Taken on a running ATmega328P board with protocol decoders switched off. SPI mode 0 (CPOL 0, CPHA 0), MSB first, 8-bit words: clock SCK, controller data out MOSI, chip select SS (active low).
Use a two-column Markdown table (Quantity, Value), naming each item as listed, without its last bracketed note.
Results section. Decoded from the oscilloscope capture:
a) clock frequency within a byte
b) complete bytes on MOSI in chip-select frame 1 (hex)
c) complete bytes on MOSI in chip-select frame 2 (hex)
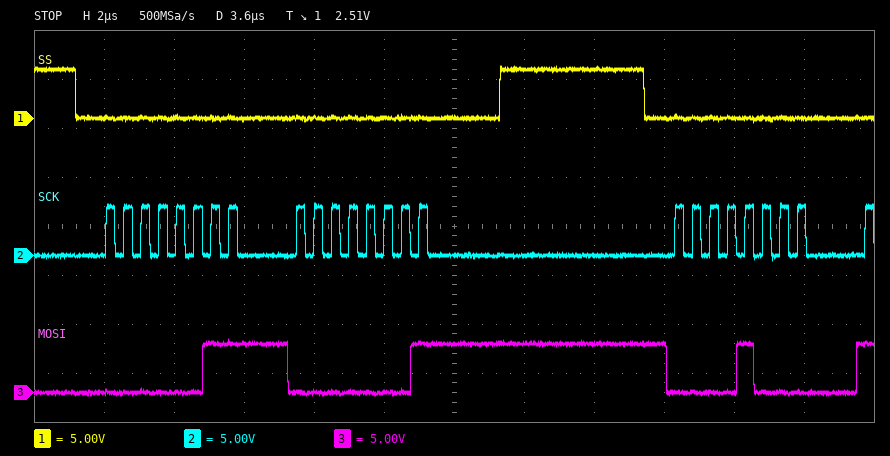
| Quantity | Value |
|---|---|
| clock frequency within a byte | 2 MHz |
| complete bytes on MOSI in chip-select frame 1 | 03 01 |
| complete bytes on MOSI in chip-select frame 2 | 08 |
